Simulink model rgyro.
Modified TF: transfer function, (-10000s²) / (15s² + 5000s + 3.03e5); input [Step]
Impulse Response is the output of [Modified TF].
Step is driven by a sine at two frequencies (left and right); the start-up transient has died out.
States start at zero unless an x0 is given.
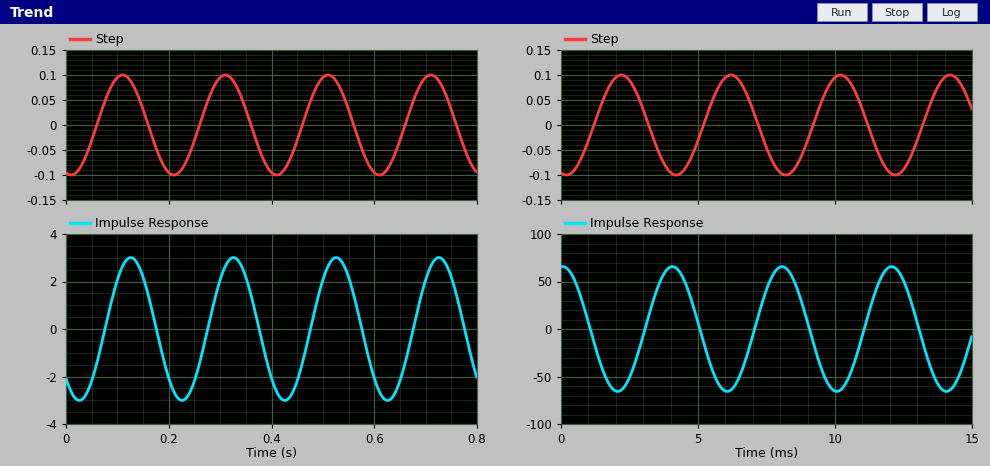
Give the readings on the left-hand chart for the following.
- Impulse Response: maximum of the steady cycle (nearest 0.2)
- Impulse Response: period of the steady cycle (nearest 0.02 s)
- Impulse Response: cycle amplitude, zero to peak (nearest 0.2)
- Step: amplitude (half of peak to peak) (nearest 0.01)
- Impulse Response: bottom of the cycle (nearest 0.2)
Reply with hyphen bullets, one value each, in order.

- 3.0
- 0.20 s
- 3.0
- 0.10
- -3.0
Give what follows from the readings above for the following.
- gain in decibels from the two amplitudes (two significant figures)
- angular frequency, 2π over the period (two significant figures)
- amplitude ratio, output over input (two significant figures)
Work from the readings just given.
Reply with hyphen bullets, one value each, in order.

- 30 dB
- 31 rad/s
- 30
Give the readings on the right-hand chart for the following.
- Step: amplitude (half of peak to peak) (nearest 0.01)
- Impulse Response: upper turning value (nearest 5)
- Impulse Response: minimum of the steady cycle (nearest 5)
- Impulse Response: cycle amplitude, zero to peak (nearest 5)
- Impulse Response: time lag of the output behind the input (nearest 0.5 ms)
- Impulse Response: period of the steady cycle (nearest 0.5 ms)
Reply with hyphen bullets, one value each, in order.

- 0.10
- 65
- -65
- 65
- 2.0 ms
- 4.0 ms
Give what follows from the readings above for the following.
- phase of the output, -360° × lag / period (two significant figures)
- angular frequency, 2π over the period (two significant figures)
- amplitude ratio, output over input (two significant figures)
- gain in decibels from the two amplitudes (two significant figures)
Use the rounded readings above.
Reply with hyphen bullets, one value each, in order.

- -180°
- 1.6 rad/ms
- 650
- 56 dB
